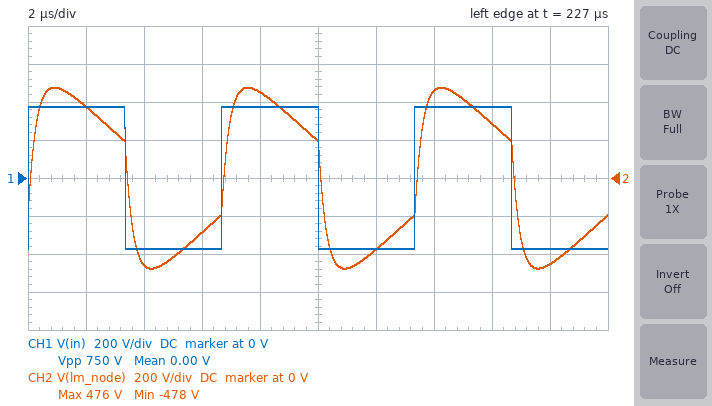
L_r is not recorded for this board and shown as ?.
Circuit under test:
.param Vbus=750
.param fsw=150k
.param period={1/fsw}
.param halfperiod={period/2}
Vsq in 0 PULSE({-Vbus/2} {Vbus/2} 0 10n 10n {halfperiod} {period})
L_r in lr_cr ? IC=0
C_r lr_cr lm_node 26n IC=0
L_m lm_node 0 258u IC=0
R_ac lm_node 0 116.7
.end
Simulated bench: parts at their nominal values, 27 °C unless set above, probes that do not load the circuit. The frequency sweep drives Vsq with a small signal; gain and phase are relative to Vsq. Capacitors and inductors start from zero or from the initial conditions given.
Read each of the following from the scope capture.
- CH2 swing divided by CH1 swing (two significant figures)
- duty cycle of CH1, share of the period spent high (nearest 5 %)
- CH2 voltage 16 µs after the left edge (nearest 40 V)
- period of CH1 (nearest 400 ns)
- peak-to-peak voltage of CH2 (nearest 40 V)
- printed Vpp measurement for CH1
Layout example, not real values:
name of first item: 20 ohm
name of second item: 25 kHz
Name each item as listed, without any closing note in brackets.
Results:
CH2 swing divided by CH1 swing: 1.3
duty cycle of CH1, share of the period spent high: 50 %
CH2 voltage 16 µs after the left edge: 280 V
period of CH1: 6.8 µs
peak-to-peak voltage of CH2: 960 V
printed Vpp measurement for CH1: 750 V
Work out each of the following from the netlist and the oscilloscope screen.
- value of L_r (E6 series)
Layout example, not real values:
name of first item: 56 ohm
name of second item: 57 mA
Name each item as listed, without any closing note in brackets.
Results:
value of L_r: 33 µH
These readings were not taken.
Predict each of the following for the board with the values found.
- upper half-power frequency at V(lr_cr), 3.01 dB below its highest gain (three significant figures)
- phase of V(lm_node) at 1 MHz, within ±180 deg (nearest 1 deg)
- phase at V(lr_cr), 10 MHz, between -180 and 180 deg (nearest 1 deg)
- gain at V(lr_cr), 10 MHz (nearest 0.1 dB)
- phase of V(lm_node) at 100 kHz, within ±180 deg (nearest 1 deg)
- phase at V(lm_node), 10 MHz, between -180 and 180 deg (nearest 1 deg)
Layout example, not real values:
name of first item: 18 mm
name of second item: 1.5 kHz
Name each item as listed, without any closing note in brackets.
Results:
upper half-power frequency at V(lr_cr), 3.01 dB below its highest gain: 374 kHz
phase of V(lm_node) at 1 MHz, within ±180 deg: -57 deg
phase at V(lr_cr), 10 MHz, between -180 and 180 deg: -87 deg
gain at V(lr_cr), 10 MHz: -25.0 dB
phase of V(lm_node) at 100 kHz, within ±180 deg: 25 deg
phase at V(lm_node), 10 MHz, between -180 and 180 deg: -86 deg
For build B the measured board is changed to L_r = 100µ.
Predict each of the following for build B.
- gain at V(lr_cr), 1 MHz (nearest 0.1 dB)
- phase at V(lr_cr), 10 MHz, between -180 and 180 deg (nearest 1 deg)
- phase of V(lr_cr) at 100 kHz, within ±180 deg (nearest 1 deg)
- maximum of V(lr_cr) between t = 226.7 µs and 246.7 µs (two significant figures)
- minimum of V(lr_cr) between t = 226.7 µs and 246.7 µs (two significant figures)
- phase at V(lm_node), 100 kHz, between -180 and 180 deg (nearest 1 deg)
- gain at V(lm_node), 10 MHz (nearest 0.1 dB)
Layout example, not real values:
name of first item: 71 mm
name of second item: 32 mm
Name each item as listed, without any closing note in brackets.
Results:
gain at V(lr_cr), 1 MHz: -14.8 dB
phase at V(lr_cr), 10 MHz, between -180 and 180 deg: -89 deg
phase of V(lr_cr) at 100 kHz, within ±180 deg: -41 deg
maximum of V(lr_cr) between t = 226.7 µs and 246.7 µs: 350 V
minimum of V(lr_cr) between t = 226.7 µs and 246.7 µs: -350 V
phase at V(lm_node), 100 kHz, between -180 and 180 deg: -1 deg
gain at V(lm_node), 10 MHz: -34.6 dB
